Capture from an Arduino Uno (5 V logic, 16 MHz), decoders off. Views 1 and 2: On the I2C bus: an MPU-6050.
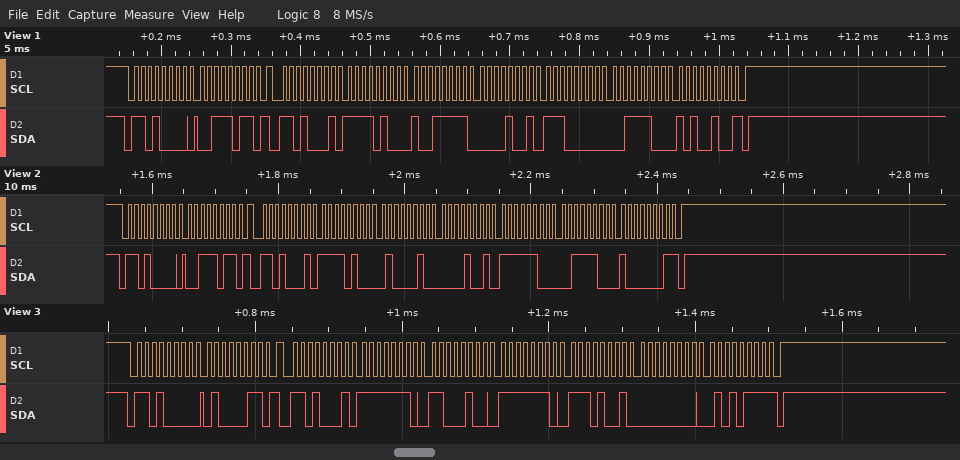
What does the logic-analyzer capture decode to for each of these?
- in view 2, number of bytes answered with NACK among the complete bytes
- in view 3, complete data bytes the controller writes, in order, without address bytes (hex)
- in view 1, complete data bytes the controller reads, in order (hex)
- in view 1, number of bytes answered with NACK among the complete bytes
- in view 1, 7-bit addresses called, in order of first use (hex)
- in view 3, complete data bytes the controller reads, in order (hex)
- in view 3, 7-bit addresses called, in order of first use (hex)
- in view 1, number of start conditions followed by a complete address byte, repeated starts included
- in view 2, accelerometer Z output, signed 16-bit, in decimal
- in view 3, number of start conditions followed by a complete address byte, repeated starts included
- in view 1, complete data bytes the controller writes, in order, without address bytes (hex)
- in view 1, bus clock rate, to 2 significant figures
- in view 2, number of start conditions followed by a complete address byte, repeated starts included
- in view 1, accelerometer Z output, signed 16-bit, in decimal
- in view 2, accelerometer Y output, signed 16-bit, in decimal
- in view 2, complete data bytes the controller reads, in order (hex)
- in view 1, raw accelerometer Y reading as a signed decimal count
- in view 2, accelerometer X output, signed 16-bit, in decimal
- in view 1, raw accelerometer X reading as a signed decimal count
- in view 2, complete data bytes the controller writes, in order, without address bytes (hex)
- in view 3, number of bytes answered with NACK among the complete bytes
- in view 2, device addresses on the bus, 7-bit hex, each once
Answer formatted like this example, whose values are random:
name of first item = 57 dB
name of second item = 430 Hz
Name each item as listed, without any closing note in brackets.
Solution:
in view 2, number of bytes answered with NACK among the complete bytes = 1
in view 3, complete data bytes the controller writes, in order, without address bytes = 43
in view 1, complete data bytes the controller reads, in order = F4 9F 09 E0 3C A4
in view 1, number of bytes answered with NACK among the complete bytes = 1
in view 1, 7-bit addresses called, in order of first use = 0x68
in view 3, complete data bytes the controller reads, in order = FE C4 FE E9 00 57
in view 3, 7-bit addresses called, in order of first use = 0x68
in view 1, number of start conditions followed by a complete address byte, repeated starts included = 2
in view 2, accelerometer Z output, signed 16-bit, in decimal = 15489
in view 3, number of start conditions followed by a complete address byte, repeated starts included = 2
in view 1, complete data bytes the controller writes, in order, without address bytes = 3B
in view 1, bus clock rate, to 2 significant figures = 100 kHz
in view 2, number of start conditions followed by a complete address byte, repeated starts included = 2
in view 1, accelerometer Z output, signed 16-bit, in decimal = 15524
in view 2, accelerometer Y output, signed 16-bit, in decimal = 2556
in view 2, complete data bytes the controller reads, in order = F4 42 09 FC 3C 81
in view 1, raw accelerometer Y reading as a signed decimal count = 2528
in view 2, accelerometer X output, signed 16-bit, in decimal = -3006
in view 1, raw accelerometer X reading as a signed decimal count = -2913
in view 2, complete data bytes the controller writes, in order, without address bytes = 3B
in view 3, number of bytes answered with NACK among the complete bytes = 1
in view 2, device addresses on the bus, 7-bit hex, each once = 0x68
